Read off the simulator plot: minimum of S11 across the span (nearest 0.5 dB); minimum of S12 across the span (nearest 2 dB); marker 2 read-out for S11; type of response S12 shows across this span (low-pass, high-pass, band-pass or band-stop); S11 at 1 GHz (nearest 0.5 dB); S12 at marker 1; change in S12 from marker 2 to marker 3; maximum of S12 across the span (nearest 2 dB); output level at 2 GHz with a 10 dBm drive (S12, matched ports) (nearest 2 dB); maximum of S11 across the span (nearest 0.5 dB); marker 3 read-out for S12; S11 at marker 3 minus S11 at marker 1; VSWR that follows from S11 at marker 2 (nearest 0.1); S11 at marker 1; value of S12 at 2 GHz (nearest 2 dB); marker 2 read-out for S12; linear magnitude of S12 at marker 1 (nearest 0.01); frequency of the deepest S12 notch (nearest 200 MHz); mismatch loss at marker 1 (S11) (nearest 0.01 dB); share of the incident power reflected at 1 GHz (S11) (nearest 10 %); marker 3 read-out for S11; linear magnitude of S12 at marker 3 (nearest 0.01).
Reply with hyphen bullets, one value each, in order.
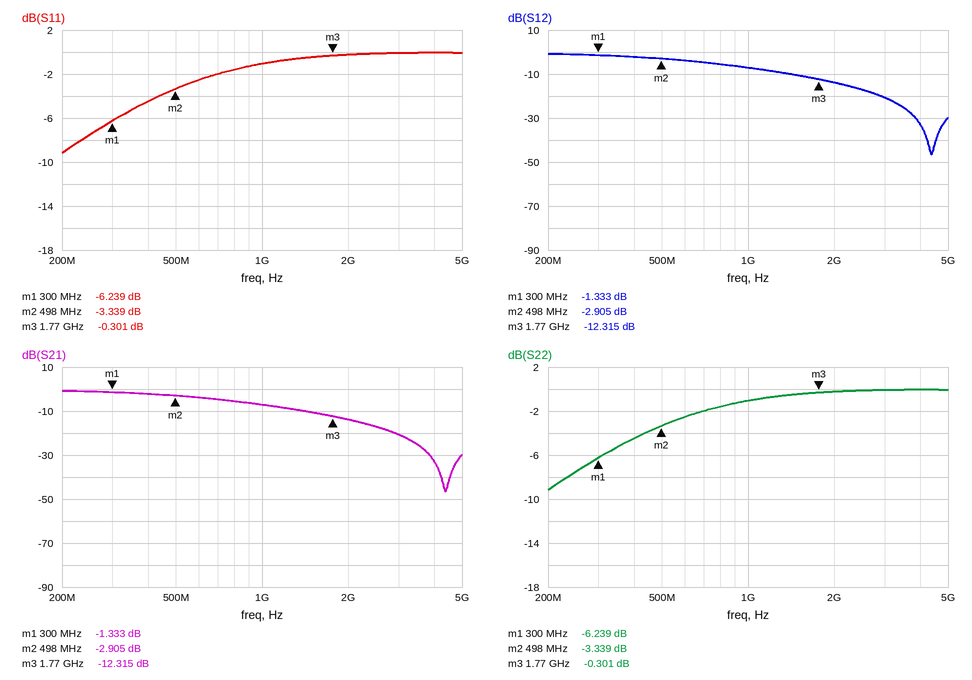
- -9.0 dB
- -46 dB
- -3.339 dB
- low-pass
- -1.0 dB
- -1.333 dB
- -9.410 dB
- 0 dB
- -4 dBm
- 0.0 dB
- -12.315 dB
- 5.938 dB
- 5.3
- -6.239 dB
- -14 dB
- -2.905 dB
- 0.86
- 4.4 GHz
- 1.18 dB
- 80 %
- -0.301 dB
- 0.24
